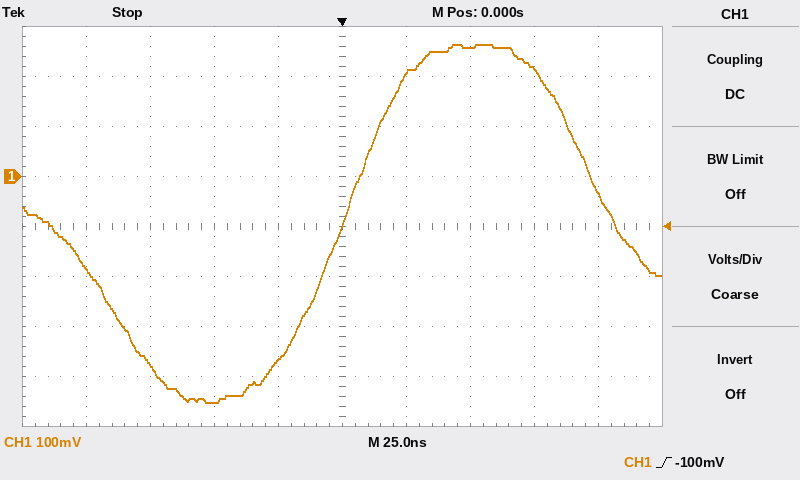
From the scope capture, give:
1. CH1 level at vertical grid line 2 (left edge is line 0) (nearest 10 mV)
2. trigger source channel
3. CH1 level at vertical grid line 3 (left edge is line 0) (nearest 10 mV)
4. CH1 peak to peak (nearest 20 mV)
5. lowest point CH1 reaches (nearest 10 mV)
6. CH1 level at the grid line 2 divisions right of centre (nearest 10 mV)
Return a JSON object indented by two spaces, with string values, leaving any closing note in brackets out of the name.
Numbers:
{
  "CH1 level at vertical grid line 2 (left edge is line 0)": "-380 mV",
  "trigger source channel": "CH1",
  "CH1 level at vertical grid line 3 (left edge is line 0)": "-450 mV",
  "CH1 peak to peak": "720 mV",
  "lowest point CH1 reaches": "-450 mV",
  "CH1 level at the grid line 2 divisions right of centre": "260 mV"
}
